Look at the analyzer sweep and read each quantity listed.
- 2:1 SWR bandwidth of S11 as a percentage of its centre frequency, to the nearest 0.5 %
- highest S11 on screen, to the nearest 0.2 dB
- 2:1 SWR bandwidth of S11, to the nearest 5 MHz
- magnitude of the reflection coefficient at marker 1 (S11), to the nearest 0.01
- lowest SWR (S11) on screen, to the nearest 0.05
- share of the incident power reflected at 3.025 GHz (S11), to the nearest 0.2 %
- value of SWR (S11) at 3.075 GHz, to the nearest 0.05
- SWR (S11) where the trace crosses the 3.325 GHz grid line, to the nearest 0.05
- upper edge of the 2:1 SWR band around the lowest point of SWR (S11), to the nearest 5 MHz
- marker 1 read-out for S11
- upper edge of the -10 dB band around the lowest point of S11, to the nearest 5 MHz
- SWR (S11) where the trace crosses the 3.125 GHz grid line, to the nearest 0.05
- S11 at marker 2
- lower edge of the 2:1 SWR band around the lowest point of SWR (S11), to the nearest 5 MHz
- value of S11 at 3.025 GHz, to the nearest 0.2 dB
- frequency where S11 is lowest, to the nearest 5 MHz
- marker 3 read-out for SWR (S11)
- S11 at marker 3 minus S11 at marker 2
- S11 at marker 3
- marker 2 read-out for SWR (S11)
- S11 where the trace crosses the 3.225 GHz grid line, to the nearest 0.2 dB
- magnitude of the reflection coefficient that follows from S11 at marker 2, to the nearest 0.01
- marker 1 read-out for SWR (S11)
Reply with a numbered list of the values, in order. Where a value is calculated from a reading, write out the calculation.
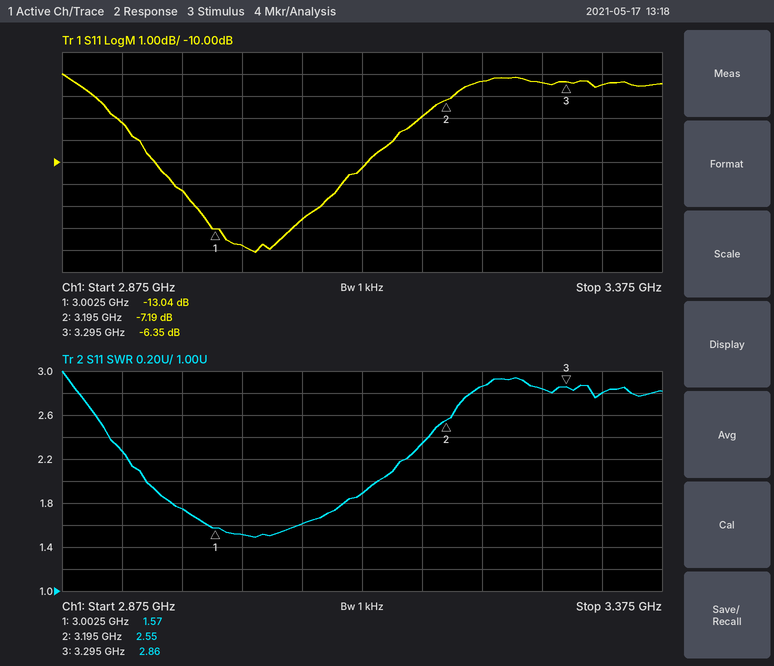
1. 195 MHz / 3.0425 GHz ≈ 6.41 %, so 6.5 % to the nearest 0.5 %
2. -6.0 dB
3. 3.140 GHz − 2.945 GHz = 195 MHz
4. 10^(-13.04/20) ≈ 0.22
5. 1.50
6. 10^(-13.8/10) ≈ 4.2 %
7. 1.60
8. 2.80
9. 3.140 GHz
10. -13.04 dB
11. 3.130 GHz
12. 1.90
13. -7.19 dB
14. 2.945 GHz
15. -13.8 dB
16. 3.035 GHz
17. 2.86
18. -6.35 − (-7.19) = 0.84 dB
19. -6.35 dB
20. 2.55
21. -6.4 dB
22. 10^(-7.19/20) ≈ 0.44
23. 1.57
